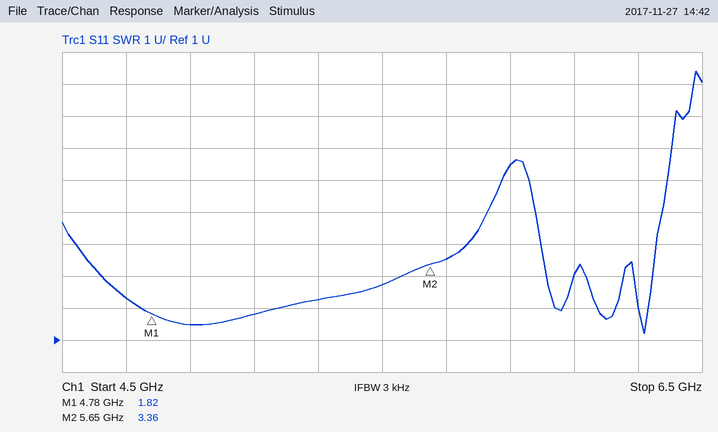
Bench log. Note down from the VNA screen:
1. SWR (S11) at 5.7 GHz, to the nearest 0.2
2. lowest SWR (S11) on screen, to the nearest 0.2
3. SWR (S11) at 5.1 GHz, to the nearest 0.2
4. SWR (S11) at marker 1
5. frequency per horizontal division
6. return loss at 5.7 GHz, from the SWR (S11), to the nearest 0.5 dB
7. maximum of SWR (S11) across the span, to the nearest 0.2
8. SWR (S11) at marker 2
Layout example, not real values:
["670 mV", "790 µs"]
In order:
["3.6", "1.2", "1.8", "1.82", "200 MHz", "5.0 dB", "9.4", "3.36"]
